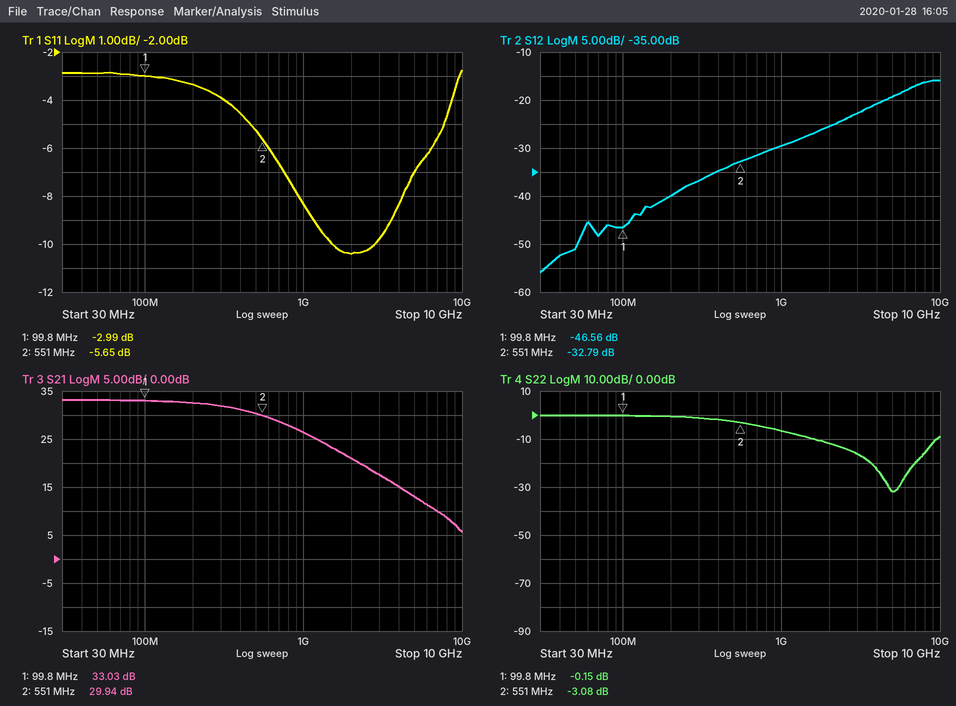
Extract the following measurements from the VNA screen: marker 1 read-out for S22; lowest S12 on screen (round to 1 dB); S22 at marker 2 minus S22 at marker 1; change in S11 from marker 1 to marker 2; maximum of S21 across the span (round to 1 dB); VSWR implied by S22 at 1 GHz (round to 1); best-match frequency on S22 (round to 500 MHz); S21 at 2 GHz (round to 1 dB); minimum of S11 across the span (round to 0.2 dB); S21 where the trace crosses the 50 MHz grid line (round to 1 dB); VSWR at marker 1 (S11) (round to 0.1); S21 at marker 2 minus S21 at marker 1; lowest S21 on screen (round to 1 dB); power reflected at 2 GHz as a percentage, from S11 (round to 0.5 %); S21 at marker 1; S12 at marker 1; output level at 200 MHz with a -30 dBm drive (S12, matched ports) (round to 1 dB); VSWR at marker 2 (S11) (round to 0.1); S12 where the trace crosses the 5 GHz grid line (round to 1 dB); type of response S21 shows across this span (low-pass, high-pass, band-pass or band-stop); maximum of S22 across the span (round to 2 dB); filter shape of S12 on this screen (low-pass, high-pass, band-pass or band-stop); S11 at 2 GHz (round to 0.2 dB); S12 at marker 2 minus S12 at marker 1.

-0.15 dB
-56 dB
-2.93 dB
-2.66 dB
33 dB
3
5.0 GHz
21 dB
-10.4 dB
33 dB
5.9
-3.09 dB
6 dB
9.0 %
33.03 dB
-46.56 dB
-70 dBm
3.2
-19 dB
low-pass
0 dB
high-pass
-10.4 dB
13.77 dB
